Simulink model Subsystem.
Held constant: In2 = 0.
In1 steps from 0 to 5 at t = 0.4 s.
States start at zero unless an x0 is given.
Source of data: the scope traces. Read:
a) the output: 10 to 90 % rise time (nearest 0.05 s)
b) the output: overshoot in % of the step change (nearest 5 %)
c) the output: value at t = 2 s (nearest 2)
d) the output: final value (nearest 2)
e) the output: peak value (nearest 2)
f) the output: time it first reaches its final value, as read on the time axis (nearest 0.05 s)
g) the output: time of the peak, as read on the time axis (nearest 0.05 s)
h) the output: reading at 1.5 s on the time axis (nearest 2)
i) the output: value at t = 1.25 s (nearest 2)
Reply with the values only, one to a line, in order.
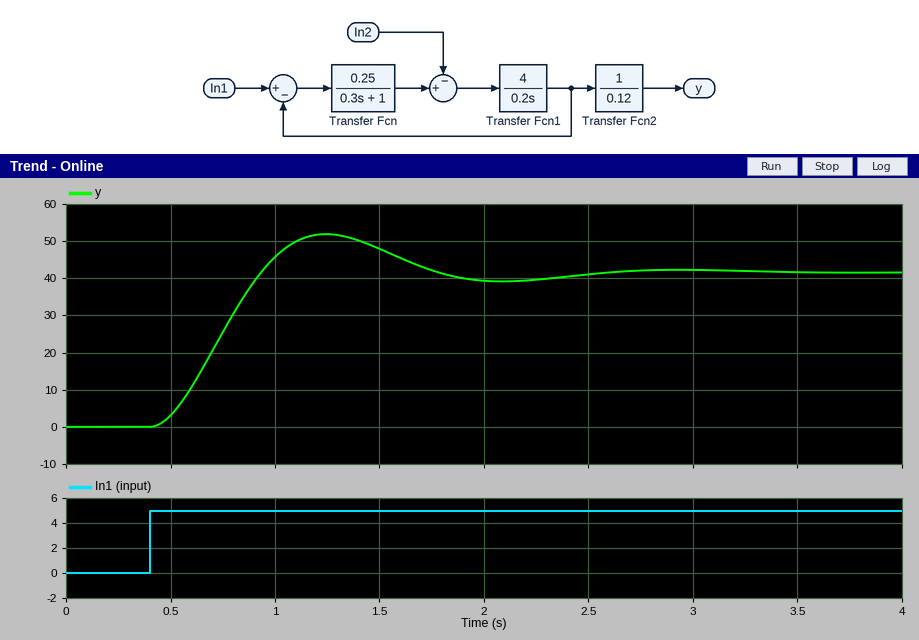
0.35 s
25 %
40
42
52
0.95 s
1.25 s
48
52
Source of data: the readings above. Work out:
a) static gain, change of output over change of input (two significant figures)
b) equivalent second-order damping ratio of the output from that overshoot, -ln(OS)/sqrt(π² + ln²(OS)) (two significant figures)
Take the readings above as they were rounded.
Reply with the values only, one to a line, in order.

8.4
0.40
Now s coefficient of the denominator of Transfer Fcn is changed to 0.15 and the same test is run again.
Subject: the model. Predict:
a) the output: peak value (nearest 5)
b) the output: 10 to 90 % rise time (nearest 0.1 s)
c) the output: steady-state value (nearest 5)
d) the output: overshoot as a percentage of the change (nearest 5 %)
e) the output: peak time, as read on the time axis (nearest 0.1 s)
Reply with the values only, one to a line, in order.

45
0.3 s
40
10 %
1.1 s
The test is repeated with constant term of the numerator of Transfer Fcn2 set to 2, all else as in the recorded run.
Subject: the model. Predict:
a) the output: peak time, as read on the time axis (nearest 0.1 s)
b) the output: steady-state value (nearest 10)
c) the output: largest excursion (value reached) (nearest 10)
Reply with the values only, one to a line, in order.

1.2 s
80
100
